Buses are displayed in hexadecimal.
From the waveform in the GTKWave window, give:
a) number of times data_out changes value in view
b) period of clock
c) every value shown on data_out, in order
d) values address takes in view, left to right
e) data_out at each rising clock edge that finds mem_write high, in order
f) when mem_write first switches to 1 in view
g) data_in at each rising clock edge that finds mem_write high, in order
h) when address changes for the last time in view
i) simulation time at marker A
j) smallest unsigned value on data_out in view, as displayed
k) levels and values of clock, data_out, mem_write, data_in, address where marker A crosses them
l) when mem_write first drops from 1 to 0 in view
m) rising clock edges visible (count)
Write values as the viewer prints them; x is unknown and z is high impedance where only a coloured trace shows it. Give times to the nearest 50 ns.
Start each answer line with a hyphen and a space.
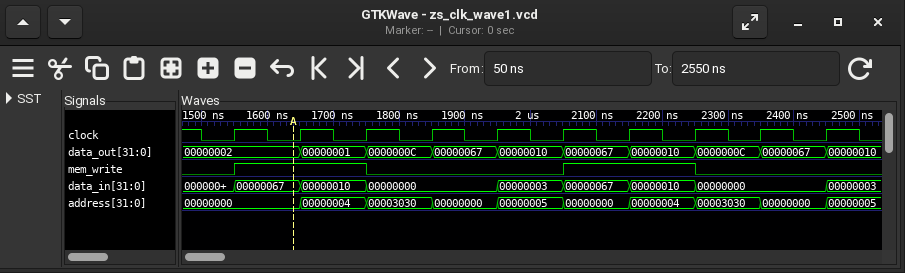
- 9
- 100 ns
- 00000002, 00000001, 0000000C, 00000067, 00000010, 00000067, 00000010, 0000000C, 00000067, 00000010
- 00000000, 00000004, 00003030, 00000000, 00000005, 00000000, 00000004, 00003030, 00000000, 00000005
- 00000002, 00000001, 00000067, 00000010
- 1550 ns
- 00000067, 00000010, 00000067, 00000010
- 2450 ns
- 1650 ns
- 00000001
- clock=0, data_out=00000002, mem_write=1, data_in=00000067, address=00000000
- 1750 ns
- 10
